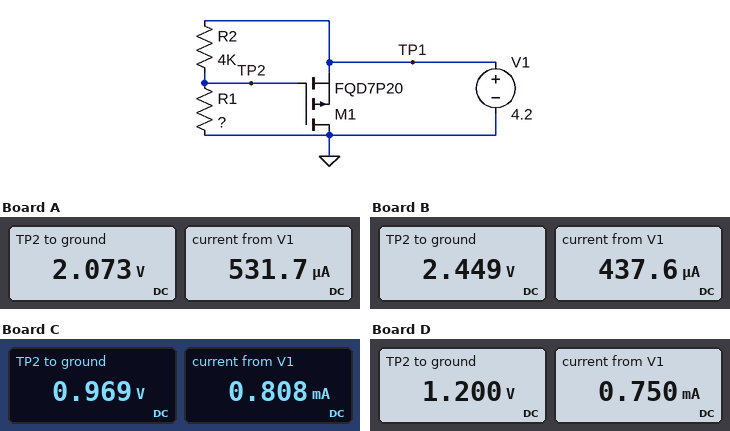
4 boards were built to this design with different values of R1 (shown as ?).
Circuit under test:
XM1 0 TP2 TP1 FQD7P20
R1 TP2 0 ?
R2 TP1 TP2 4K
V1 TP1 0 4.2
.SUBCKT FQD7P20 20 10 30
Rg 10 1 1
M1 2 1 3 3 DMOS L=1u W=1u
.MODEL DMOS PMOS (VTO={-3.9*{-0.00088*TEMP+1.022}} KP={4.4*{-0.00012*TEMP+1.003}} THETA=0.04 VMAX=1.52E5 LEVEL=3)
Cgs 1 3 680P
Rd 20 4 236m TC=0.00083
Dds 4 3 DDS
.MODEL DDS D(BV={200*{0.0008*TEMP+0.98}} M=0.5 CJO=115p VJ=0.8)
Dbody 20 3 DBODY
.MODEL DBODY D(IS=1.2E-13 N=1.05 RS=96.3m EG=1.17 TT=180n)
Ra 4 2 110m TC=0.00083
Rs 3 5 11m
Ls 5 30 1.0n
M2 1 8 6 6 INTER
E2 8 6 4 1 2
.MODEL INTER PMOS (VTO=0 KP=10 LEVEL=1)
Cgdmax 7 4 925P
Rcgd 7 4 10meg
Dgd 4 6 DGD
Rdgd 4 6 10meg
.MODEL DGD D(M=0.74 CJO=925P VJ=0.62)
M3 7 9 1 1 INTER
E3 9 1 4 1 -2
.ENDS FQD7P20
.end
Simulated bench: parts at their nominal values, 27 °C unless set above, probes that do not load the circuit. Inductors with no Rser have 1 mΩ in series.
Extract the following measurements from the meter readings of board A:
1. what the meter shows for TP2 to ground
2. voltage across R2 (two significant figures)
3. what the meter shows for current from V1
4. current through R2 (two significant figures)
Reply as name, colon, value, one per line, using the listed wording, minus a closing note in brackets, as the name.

what the meter shows for TP2 to ground: 2.073 V
voltage across R2: 2.1 V
what the meter shows for current from V1: 531.7 µA
current through R2: 530 µA
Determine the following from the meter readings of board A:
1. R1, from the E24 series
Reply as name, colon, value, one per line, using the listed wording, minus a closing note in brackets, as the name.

R1, from the E24 series: 3.9 kΩ
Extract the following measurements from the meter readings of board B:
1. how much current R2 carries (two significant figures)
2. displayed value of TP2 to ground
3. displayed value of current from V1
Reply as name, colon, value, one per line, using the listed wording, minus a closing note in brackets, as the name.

how much current R2 carries: 440 µA
displayed value of TP2 to ground: 2.449 V
displayed value of current from V1: 437.6 µA
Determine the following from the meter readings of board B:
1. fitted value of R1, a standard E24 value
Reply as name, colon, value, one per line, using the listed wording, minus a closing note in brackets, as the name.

fitted value of R1, a standard E24 value: 5.6 kΩ
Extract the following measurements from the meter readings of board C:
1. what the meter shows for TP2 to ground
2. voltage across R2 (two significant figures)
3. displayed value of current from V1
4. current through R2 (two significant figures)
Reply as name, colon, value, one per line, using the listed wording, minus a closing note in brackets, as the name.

what the meter shows for TP2 to ground: 0.969 V
voltage across R2: 3.2 V
displayed value of current from V1: 0.808 mA
current through R2: 810 µA
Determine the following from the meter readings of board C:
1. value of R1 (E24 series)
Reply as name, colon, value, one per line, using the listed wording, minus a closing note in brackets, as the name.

value of R1: 1.2 kΩ
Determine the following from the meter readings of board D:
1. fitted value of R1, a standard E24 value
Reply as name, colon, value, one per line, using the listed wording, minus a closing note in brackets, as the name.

fitted value of R1, a standard E24 value: 1.6 kΩ
